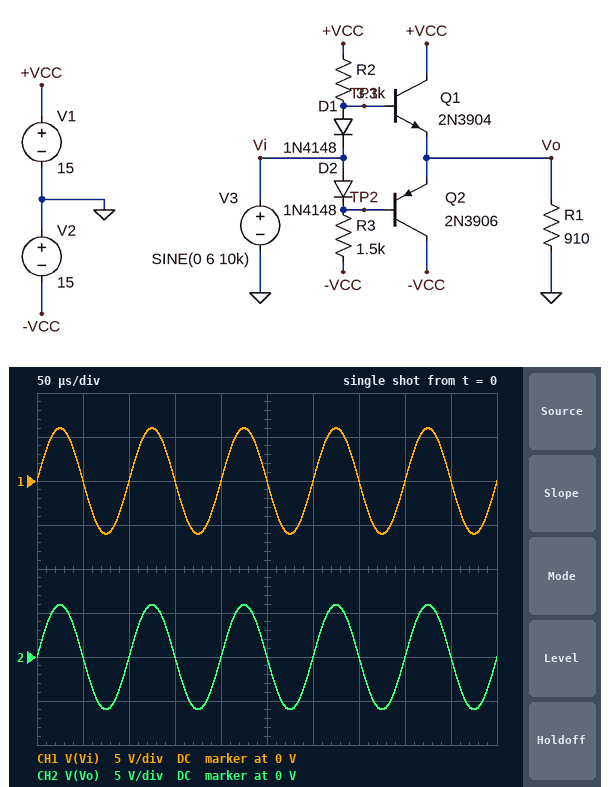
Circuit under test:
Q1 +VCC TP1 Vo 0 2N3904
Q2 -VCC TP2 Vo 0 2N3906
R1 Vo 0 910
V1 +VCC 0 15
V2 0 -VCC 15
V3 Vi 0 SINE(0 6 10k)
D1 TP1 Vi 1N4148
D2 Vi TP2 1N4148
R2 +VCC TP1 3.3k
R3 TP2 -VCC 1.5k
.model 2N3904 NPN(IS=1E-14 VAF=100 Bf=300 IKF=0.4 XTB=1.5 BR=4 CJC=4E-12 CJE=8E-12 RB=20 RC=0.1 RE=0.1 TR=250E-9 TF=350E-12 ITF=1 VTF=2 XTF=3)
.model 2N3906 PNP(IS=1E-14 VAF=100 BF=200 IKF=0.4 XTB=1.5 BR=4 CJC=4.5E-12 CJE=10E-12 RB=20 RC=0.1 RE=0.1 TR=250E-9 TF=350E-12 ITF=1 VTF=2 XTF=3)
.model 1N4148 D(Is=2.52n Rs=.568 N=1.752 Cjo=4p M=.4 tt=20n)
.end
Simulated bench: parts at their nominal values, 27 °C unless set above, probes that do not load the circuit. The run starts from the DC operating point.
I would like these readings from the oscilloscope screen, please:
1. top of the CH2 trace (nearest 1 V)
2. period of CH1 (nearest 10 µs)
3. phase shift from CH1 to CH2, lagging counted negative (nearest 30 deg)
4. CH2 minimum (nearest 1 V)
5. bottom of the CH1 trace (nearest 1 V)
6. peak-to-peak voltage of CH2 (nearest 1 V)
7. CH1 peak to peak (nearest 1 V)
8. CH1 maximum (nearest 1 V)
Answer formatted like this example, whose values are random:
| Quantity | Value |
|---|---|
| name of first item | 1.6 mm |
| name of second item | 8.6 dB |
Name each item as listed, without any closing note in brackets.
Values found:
| Quantity | Value |
|---|---|
| top of the CH2 trace | 6 V |
| period of CH1 | 100 µs |
| phase shift from CH1 to CH2, lagging counted negative | 0 deg |
| CH2 minimum | -6 V |
| bottom of the CH1 trace | -6 V |
| peak-to-peak voltage of CH2 | 12 V |
| CH1 peak to peak | 12 V |
| CH1 maximum | 6 V |
